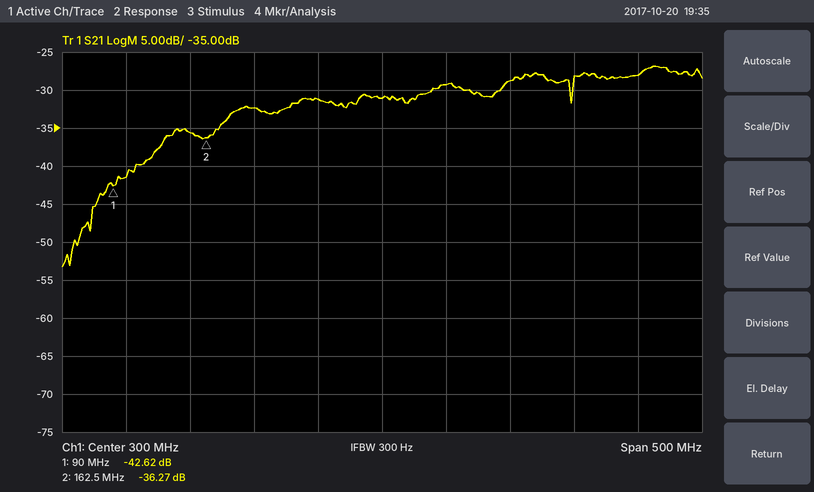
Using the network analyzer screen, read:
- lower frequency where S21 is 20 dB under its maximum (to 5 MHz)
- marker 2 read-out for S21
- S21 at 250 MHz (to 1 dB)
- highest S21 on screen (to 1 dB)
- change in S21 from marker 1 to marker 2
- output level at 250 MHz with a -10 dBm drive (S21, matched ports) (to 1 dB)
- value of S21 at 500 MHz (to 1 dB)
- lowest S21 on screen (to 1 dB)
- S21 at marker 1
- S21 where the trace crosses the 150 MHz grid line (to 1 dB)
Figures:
75 MHz
-36.27 dB
-31 dB
-27 dB
6.35 dB
-41 dBm
-28 dB
-53 dB
-42.62 dB
-36 dB
